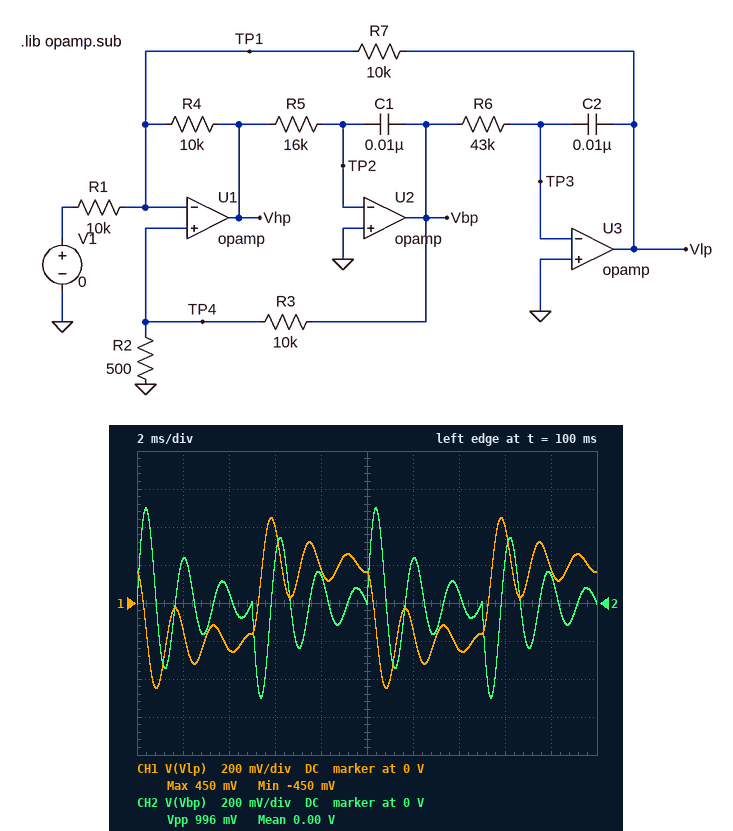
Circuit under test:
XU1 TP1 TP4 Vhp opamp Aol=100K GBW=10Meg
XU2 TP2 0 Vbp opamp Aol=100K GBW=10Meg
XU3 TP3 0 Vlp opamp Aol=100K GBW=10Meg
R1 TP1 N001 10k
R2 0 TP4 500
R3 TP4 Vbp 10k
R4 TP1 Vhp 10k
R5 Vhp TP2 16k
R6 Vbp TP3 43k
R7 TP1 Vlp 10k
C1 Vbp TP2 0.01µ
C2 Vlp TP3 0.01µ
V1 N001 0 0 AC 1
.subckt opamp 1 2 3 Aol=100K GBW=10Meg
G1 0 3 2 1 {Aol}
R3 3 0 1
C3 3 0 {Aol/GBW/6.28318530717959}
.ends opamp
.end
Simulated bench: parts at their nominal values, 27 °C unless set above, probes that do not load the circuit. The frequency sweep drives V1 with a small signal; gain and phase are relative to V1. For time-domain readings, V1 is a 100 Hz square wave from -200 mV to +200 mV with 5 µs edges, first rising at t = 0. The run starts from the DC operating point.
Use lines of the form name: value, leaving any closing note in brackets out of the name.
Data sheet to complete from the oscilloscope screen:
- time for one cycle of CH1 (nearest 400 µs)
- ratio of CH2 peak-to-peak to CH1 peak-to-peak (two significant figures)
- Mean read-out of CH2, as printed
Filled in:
time for one cycle of CH1: 10.0 ms
ratio of CH2 peak-to-peak to CH1 peak-to-peak: 1.1
Mean read-out of CH2, as printed: 0.00 V
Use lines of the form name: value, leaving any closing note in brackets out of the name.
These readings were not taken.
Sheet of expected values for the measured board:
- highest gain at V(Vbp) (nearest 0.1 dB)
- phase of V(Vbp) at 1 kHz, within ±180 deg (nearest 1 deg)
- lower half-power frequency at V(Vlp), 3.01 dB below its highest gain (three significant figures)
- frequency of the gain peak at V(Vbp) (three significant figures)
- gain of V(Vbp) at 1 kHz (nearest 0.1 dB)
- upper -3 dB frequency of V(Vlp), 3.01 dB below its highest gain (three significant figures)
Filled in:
highest gain at V(Vbp): 16.9 dB
phase of V(Vbp) at 1 kHz, within ±180 deg: -77 deg
lower half-power frequency at V(Vlp), 3.01 dB below its highest gain: 522 Hz
frequency of the gain peak at V(Vbp): 607 Hz
gain of V(Vbp) at 1 kHz: 3.7 dB
upper -3 dB frequency of V(Vlp), 3.01 dB below its highest gain: 666 Hz
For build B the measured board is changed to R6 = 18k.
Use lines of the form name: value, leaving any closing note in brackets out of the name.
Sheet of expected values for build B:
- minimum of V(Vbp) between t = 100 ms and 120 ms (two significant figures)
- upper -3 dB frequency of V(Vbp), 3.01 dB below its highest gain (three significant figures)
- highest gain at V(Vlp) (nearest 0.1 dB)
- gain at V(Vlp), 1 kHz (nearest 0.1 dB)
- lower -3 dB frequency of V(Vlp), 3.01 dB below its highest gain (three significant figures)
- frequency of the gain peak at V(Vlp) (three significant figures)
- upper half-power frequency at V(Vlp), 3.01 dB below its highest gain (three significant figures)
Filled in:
minimum of V(Vbp) between t = 100 ms and 120 ms: -400 mV
upper -3 dB frequency of V(Vbp), 3.01 dB below its highest gain: 1.01 kHz
highest gain at V(Vlp): 16.4 dB
gain at V(Vlp), 1 kHz: 13.5 dB
lower -3 dB frequency of V(Vlp), 3.01 dB below its highest gain: 858 Hz
frequency of the gain peak at V(Vlp): 932 Hz
upper half-power frequency at V(Vlp), 3.01 dB below its highest gain: 1.00 kHz
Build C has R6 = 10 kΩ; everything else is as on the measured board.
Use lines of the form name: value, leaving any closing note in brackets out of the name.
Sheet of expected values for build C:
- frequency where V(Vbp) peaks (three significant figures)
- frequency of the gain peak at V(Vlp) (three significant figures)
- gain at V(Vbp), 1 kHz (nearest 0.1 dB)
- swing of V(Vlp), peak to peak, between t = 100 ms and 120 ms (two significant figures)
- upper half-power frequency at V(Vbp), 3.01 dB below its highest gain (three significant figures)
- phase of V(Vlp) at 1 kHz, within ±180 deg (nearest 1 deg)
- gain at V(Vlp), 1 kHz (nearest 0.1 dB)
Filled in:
frequency where V(Vbp) peaks: 1.26 kHz
frequency of the gain peak at V(Vlp): 1.25 kHz
gain at V(Vbp), 1 kHz: 4.4 dB
swing of V(Vlp), peak to peak, between t = 100 ms and 120 ms: 1.1 V
upper half-power frequency at V(Vbp), 3.01 dB below its highest gain: 1.33 kHz
phase of V(Vlp) at 1 kHz, within ±180 deg: 166 deg
gain at V(Vlp), 1 kHz: 8.4 dB
